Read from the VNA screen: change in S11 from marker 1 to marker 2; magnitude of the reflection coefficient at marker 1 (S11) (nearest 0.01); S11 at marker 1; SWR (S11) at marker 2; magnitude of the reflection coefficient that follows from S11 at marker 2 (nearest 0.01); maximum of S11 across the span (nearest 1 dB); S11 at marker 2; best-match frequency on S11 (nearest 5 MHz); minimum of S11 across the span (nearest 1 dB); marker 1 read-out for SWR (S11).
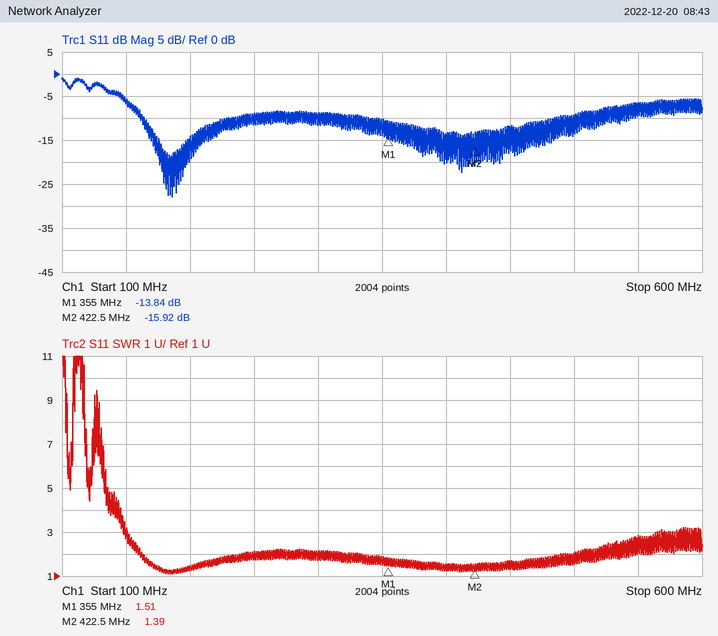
-2.08 dB
0.20
-13.84 dB
1.39
0.16
-1 dB
-15.92 dB
185 MHz
-28 dB
1.51
